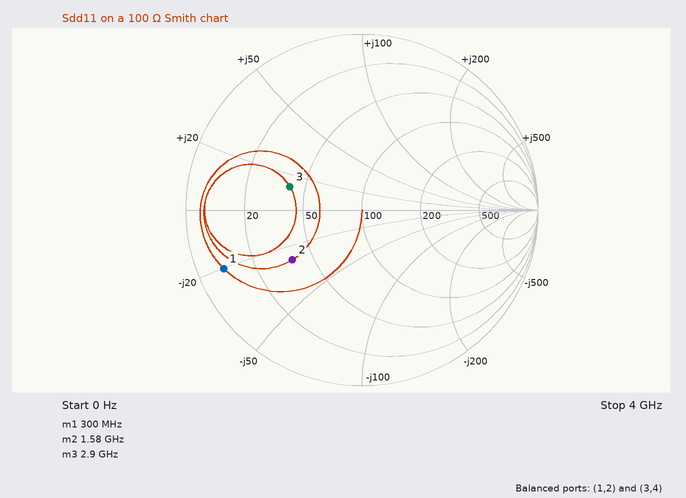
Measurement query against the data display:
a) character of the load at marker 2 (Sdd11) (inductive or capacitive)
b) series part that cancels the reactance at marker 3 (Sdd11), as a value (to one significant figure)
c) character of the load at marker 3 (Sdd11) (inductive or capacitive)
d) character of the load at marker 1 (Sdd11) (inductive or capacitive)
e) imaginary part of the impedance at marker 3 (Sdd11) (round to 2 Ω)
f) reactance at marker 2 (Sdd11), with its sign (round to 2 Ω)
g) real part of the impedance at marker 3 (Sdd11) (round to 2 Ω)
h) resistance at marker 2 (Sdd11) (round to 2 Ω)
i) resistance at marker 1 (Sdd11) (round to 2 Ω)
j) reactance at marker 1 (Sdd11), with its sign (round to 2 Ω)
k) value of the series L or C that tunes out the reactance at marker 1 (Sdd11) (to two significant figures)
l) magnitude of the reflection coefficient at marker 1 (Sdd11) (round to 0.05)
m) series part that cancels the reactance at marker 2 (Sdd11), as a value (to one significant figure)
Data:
capacitive
4 pF
inductive
capacitive
+14 Ω
-28 Ω
40 Ω
38 Ω
8 Ω
-20 Ω
11 nH
0.85
3 nH
